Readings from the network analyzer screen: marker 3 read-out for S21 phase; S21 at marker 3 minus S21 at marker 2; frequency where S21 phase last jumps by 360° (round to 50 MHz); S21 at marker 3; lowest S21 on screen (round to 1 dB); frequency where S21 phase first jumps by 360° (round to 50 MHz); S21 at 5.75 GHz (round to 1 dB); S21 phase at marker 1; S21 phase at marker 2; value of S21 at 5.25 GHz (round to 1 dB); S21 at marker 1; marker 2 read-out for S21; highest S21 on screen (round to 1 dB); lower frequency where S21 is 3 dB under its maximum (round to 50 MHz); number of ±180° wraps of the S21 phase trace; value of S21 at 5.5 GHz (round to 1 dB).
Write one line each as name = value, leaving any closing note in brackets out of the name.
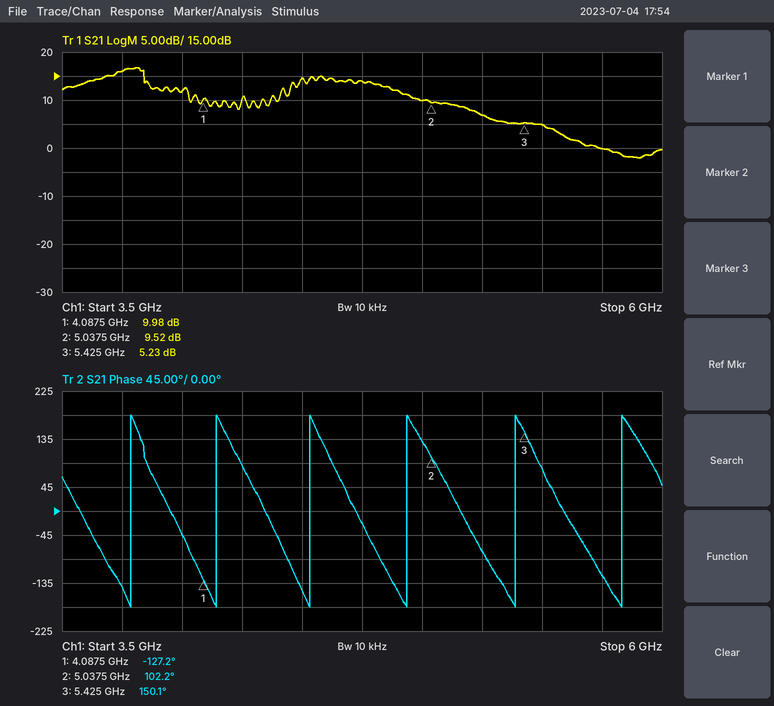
marker 3 read-out for S21 phase = 150.1°
S21 at marker 3 minus S21 at marker 2 = -4.29 dB
frequency where S21 phase last jumps by 360° = 5.85 GHz
S21 at marker 3 = 5.23 dB
lowest S21 on screen = -2 dB
frequency where S21 phase first jumps by 360° = 3.80 GHz
S21 at 5.75 GHz = 0 dB
S21 phase at marker 1 = -127.2°
S21 phase at marker 2 = 102.2°
value of S21 at 5.25 GHz = 7 dB
S21 at marker 1 = 9.98 dB
marker 2 read-out for S21 = 9.52 dB
highest S21 on screen = 17 dB
lower frequency where S21 is 3 dB under its maximum = 3.60 GHz
number of ±180° wraps of the S21 phase trace = 6
value of S21 at 5.5 GHz = 5 dB
